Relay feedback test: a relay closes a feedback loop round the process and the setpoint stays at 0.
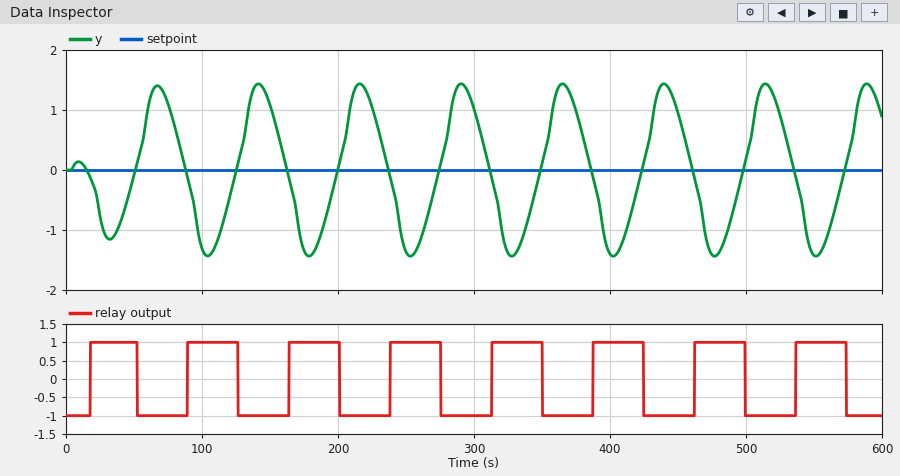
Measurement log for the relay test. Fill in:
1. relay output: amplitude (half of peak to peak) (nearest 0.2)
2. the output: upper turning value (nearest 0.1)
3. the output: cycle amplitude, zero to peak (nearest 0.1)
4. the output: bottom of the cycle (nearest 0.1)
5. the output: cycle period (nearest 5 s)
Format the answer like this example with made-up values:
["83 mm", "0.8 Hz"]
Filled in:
["1.0", "1.4", "1.4", "-1.4", "75 s"]
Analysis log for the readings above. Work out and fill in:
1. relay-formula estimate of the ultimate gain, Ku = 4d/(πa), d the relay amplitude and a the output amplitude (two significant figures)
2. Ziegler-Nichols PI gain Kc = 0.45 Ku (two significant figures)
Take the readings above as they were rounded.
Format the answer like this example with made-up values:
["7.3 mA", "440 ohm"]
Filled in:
["0.91", "0.41"]
